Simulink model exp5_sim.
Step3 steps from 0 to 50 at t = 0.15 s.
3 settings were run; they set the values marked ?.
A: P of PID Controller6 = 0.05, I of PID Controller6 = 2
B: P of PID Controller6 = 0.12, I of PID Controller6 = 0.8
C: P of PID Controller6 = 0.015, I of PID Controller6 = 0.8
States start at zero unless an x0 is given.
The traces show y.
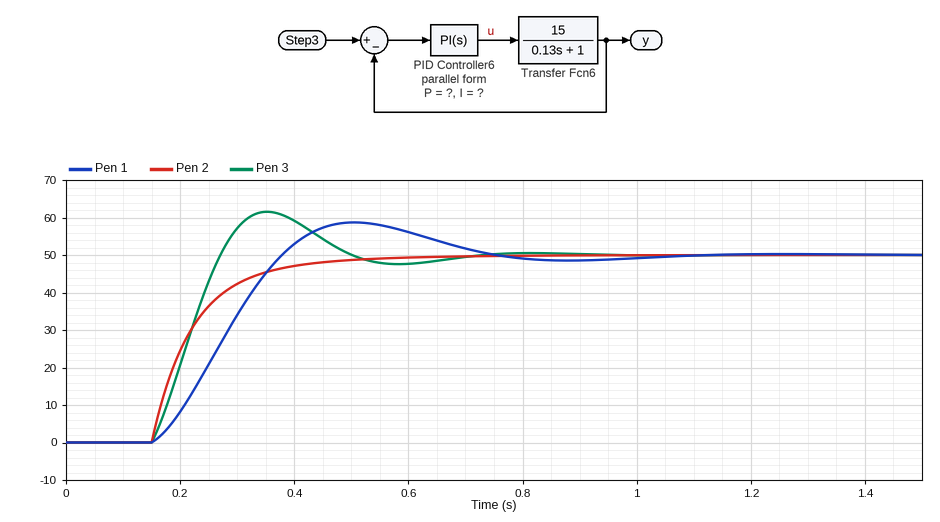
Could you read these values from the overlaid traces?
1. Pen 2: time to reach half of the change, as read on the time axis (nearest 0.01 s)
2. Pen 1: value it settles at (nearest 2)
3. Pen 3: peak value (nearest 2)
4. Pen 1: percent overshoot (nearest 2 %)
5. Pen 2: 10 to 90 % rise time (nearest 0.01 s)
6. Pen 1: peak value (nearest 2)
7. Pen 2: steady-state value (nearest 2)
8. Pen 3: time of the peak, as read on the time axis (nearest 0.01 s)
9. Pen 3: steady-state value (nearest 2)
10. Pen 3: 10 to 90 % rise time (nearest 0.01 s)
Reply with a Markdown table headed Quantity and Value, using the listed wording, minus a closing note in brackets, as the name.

| Quantity | Value |
|---|---|
| Pen 2: time to reach half of the change, as read on the time axis | 0.20 s |
| Pen 1: value it settles at | 50 |
| Pen 3: peak value | 62 |
| Pen 1: percent overshoot | 18 % |
| Pen 2: 10 to 90 % rise time | 0.18 s |
| Pen 1: peak value | 58 |
| Pen 2: steady-state value | 50 |
| Pen 3: time of the peak, as read on the time axis | 0.35 s |
| Pen 3: steady-state value | 50 |
| Pen 3: 10 to 90 % rise time | 0.09 s |
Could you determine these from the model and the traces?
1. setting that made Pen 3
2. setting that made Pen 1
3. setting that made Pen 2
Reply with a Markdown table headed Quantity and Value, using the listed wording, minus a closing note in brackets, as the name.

| Quantity | Value |
|---|---|
| setting that made Pen 3 | A |
| setting that made Pen 1 | C |
| setting that made Pen 2 | B |
